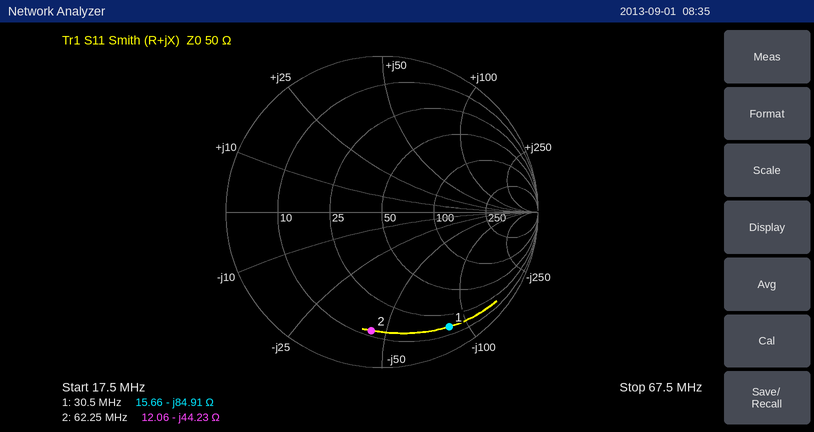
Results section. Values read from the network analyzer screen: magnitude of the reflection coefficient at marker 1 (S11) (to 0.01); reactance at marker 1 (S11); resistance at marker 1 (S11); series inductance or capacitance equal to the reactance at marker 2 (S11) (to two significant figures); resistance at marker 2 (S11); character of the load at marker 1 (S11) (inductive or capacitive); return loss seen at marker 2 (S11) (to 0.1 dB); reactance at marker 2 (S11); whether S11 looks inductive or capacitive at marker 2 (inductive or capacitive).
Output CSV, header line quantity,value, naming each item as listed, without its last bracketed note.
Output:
quantity,value
magnitude of the reflection coefficient at marker 1 (S11),0.85
reactance at marker 1,-84.91 Ω
resistance at marker 1,15.66 Ω
series inductance or capacitance equal to the reactance at marker 2 (S11),58 pF
resistance at marker 2,12.06 Ω
character of the load at marker 1 (S11),capacitive
return loss seen at marker 2 (S11),2.3 dB
reactance at marker 2,-44.23 Ω
whether S11 looks inductive or capacitive at marker 2,capacitive
